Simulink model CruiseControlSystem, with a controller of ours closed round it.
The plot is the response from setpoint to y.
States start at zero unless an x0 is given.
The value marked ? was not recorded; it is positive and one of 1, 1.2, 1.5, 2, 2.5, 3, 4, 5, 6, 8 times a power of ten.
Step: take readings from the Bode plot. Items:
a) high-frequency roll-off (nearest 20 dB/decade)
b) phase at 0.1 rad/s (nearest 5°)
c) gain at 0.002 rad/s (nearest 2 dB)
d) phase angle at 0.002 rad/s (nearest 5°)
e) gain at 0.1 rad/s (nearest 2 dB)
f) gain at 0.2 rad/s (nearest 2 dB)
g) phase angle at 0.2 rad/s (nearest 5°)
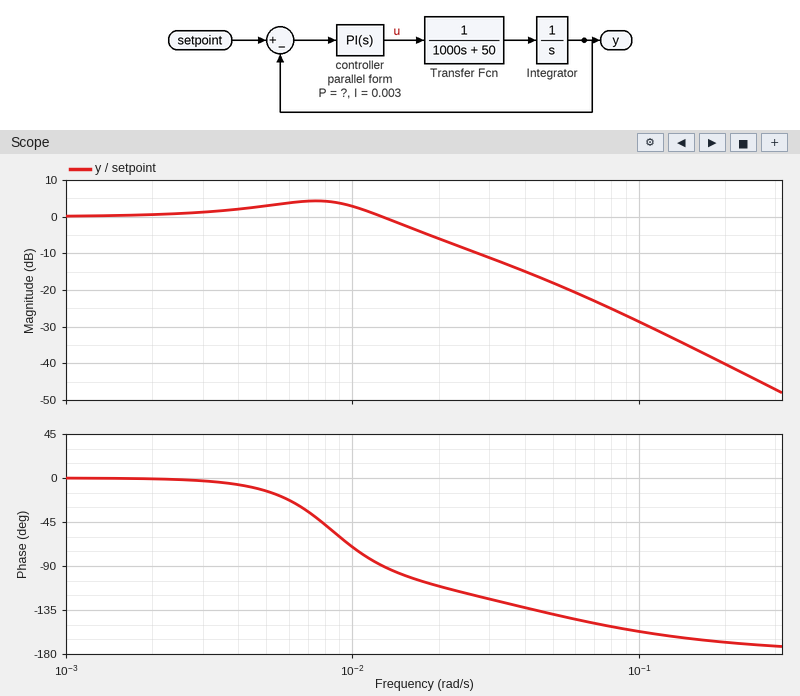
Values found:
-40 dB/decade
-155°
0 dB
0°
-28 dB
-40 dB
-170°
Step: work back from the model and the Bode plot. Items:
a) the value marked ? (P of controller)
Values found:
0.4
